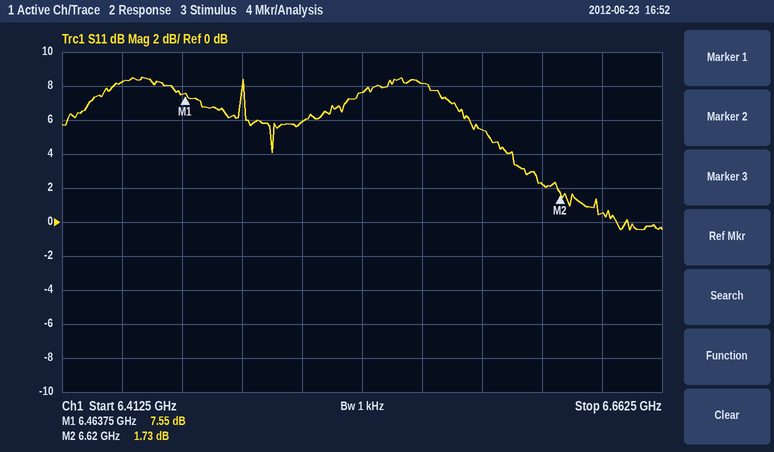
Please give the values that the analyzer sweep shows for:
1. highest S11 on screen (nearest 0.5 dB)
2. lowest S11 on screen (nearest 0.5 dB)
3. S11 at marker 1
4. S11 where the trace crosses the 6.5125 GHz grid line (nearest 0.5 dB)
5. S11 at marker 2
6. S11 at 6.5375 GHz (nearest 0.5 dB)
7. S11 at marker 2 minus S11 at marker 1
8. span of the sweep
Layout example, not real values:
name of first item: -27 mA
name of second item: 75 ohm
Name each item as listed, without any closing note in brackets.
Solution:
highest S11 on screen: 8.5 dB
lowest S11 on screen: -0.5 dB
S11 at marker 1: 7.55 dB
S11 where the trace crosses the 6.5125 GHz grid line: 6.0 dB
S11 at marker 2: 1.73 dB
S11 at 6.5375 GHz: 7.5 dB
S11 at marker 2 minus S11 at marker 1: -5.82 dB
span of the sweep: 250 MHz
